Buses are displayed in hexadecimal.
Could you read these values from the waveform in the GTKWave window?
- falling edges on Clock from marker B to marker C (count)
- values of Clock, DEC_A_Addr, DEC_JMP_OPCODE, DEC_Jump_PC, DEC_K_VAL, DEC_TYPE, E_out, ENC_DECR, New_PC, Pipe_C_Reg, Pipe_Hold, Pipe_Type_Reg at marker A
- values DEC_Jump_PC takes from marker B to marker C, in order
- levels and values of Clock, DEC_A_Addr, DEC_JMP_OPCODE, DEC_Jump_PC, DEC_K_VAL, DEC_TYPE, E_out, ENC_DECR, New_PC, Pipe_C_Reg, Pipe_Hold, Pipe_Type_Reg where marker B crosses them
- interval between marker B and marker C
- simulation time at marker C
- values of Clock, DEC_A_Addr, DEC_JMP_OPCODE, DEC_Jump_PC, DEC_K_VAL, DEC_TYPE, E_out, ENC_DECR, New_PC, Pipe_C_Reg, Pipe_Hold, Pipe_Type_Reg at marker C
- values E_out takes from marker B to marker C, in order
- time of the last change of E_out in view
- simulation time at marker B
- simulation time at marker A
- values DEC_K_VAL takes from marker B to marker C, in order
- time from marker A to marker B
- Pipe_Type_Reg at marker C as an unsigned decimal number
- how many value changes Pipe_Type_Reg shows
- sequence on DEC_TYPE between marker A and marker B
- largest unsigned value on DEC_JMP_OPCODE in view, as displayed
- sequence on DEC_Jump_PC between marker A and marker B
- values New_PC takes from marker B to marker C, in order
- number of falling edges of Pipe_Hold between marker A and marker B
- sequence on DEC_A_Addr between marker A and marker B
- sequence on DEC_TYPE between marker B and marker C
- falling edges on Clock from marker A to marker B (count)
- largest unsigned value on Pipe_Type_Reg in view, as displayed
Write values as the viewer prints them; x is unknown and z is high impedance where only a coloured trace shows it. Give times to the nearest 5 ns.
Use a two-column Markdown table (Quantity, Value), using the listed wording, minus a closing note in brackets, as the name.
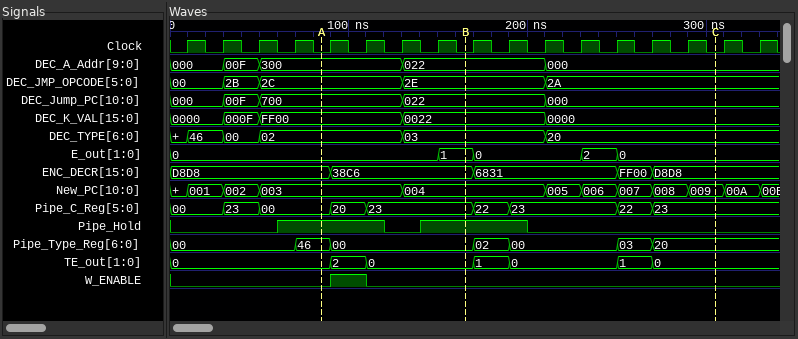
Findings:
| Quantity | Value |
|---|---|
| falling edges on Clock from marker B to marker C | 7 |
| values of Clock, DEC_A_Addr, DEC_JMP_OPCODE, DEC_Jump_PC, DEC_K_VAL, DEC_TYPE, E_out, ENC_DECR, New_PC, Pipe_C_Reg, Pipe_Hold, Pipe_Type_Reg at marker A | Clock=0, DEC_A_Addr=300, DEC_JMP_OPCODE=2C, DEC_Jump_PC=700, DEC_K_VAL=FF00, DEC_TYPE=02, E_out=0, ENC_DECR=D8D8, New_PC=003, Pipe_C_Reg=00, Pipe_Hold=1, Pipe_Type_Reg=46 |
| values DEC_Jump_PC takes from marker B to marker C, in order | 022, 000 |
| levels and values of Clock, DEC_A_Addr, DEC_JMP_OPCODE, DEC_Jump_PC, DEC_K_VAL, DEC_TYPE, E_out, ENC_DECR, New_PC, Pipe_C_Reg, Pipe_Hold, Pipe_Type_Reg where marker B crosses them | Clock=0, DEC_A_Addr=022, DEC_JMP_OPCODE=2E, DEC_Jump_PC=022, DEC_K_VAL=0022, DEC_TYPE=03, E_out=1, ENC_DECR=38C6, New_PC=004, Pipe_C_Reg=23, Pipe_Hold=1, Pipe_Type_Reg=00 |
| interval between marker B and marker C | 140 ns |
| simulation time at marker C | 305 ns |
| values of Clock, DEC_A_Addr, DEC_JMP_OPCODE, DEC_Jump_PC, DEC_K_VAL, DEC_TYPE, E_out, ENC_DECR, New_PC, Pipe_C_Reg, Pipe_Hold, Pipe_Type_Reg at marker C | Clock=0, DEC_A_Addr=000, DEC_JMP_OPCODE=2A, DEC_Jump_PC=000, DEC_K_VAL=0000, DEC_TYPE=20, E_out=0, ENC_DECR=D8D8, New_PC=009, Pipe_C_Reg=23, Pipe_Hold=0, Pipe_Type_Reg=20 |
| values E_out takes from marker B to marker C, in order | 1, 0, 2, 0 |
| time of the last change of E_out in view | 250 ns |
| simulation time at marker B | 165 ns |
| simulation time at marker A | 85 ns |
| values DEC_K_VAL takes from marker B to marker C, in order | 0022, 0000 |
| time from marker A to marker B | 80 ns |
| Pipe_Type_Reg at marker C as an unsigned decimal number | 32 |
| how many value changes Pipe_Type_Reg shows | 6 |
| sequence on DEC_TYPE between marker A and marker B | 02, 03 |
| largest unsigned value on DEC_JMP_OPCODE in view, as displayed | 2E |
| sequence on DEC_Jump_PC between marker A and marker B | 700, 022 |
| values New_PC takes from marker B to marker C, in order | 004, 005, 006, 007, 008, 009 |
| number of falling edges of Pipe_Hold between marker A and marker B | 1 |
| sequence on DEC_A_Addr between marker A and marker B | 300, 022 |
| sequence on DEC_TYPE between marker B and marker C | 03, 20 |
| falling edges on Clock from marker A to marker B | 4 |
| largest unsigned value on Pipe_Type_Reg in view, as displayed | 46 |
